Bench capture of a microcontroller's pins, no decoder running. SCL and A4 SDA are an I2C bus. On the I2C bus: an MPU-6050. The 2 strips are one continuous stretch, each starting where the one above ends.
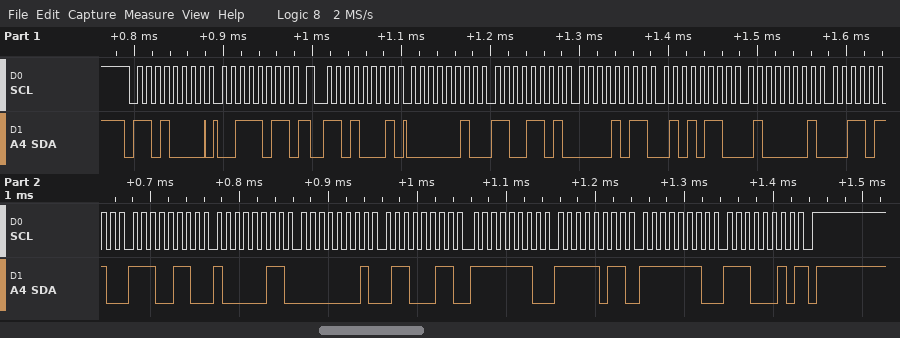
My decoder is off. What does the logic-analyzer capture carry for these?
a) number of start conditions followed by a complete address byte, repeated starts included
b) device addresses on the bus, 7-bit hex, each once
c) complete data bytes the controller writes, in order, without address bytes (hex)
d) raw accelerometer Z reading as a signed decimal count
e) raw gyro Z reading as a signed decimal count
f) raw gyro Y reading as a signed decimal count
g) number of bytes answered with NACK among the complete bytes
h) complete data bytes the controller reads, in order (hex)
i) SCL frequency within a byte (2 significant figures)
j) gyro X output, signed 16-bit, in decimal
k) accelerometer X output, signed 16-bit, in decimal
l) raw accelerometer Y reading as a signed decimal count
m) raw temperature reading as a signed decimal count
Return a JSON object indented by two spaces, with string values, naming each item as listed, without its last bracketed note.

{
  "number of start conditions followed by a complete address byte, repeated starts included": "2",
  "device addresses on the bus, 7-bit hex, each once": "0x68",
  "complete data bytes the controller writes, in order, without address bytes": "3B",
  "raw accelerometer Z reading as a signed decimal count": "16694",
  "raw gyro Z reading as a signed decimal count": "-286",
  "raw gyro Y reading as a signed decimal count": "-261",
  "number of bytes answered with NACK among the complete bytes": "1",
  "complete data bytes the controller reads, in order": "02 CD 0B 56 41 36 E6 83 01 63 FE FB FE E2",
  "SCL frequency within a byte": "100 kHz",
  "gyro X output, signed 16-bit, in decimal": "355",
  "accelerometer X output, signed 16-bit, in decimal": "717",
  "raw accelerometer Y reading as a signed decimal count": "2902",
  "raw temperature reading as a signed decimal count": "-6525"
}
